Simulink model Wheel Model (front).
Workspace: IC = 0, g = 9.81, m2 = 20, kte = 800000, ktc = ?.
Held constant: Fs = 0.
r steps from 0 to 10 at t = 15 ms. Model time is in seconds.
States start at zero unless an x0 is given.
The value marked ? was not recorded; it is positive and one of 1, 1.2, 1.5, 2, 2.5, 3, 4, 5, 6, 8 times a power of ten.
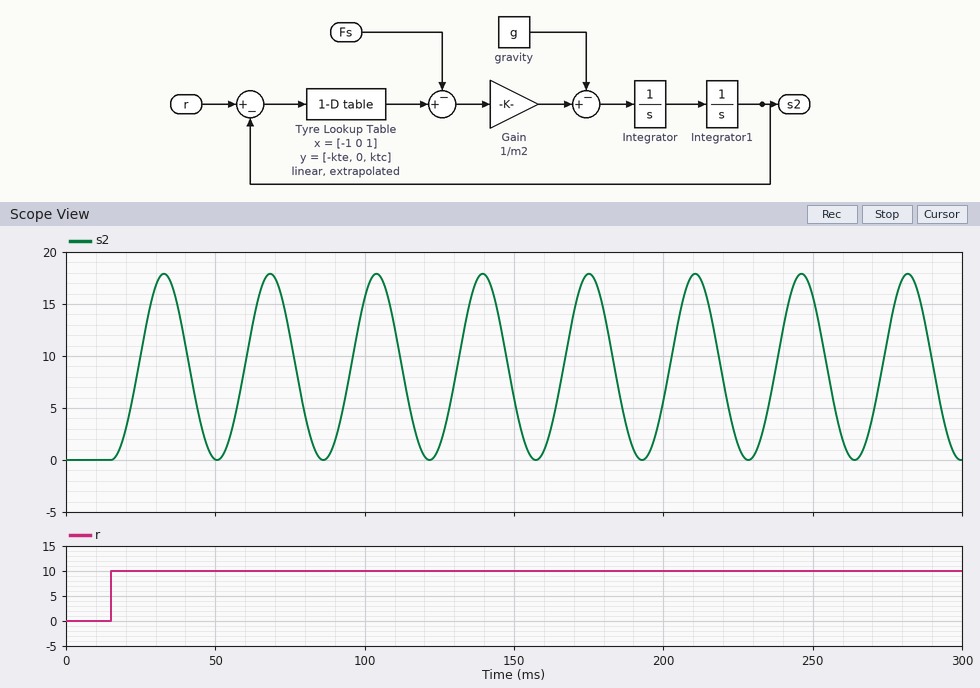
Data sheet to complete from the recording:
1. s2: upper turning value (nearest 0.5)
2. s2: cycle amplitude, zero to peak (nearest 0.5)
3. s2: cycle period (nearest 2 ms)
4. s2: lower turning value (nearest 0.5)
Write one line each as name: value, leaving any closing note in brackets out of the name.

s2: upper turning value: 18.0
s2: cycle amplitude, zero to peak: 9.0
s2: cycle period: 36 ms
s2: lower turning value: 0.0
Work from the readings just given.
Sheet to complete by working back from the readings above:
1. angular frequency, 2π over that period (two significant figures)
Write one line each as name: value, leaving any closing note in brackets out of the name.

angular frequency, 2π over that period: 0.17 rad/ms
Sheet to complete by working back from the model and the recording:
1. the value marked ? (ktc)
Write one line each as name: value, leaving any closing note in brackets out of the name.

the value marked ?: 500000
